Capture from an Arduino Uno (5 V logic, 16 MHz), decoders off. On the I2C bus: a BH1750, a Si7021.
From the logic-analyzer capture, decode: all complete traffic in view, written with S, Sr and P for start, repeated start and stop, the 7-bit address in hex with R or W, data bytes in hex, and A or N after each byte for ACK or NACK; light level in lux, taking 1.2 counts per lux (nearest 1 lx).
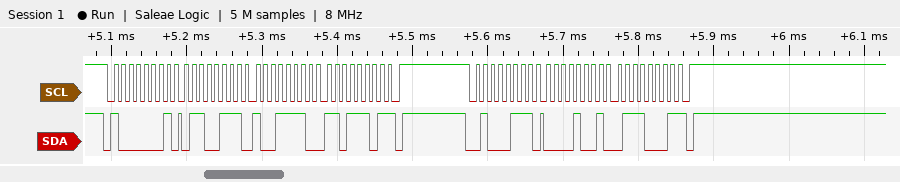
S 40R A 67 A 9E A DD N P S 23R A 09 A 71 N P
2014 lx
